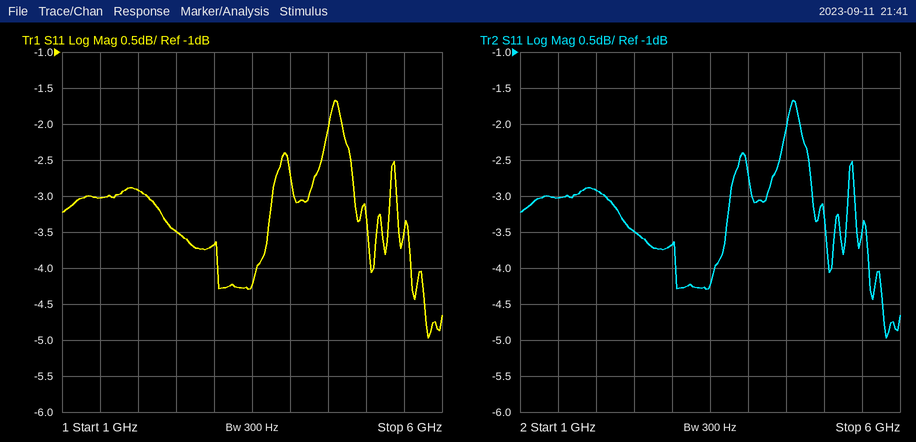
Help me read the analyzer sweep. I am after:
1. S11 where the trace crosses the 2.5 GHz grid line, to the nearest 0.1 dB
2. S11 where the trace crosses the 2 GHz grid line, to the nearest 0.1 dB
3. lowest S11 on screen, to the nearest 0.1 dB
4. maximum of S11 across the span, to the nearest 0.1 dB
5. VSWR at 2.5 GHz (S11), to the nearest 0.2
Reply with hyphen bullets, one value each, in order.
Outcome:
- -3.5 dB
- -2.9 dB
- -5.0 dB
- -1.7 dB
- 5.0
